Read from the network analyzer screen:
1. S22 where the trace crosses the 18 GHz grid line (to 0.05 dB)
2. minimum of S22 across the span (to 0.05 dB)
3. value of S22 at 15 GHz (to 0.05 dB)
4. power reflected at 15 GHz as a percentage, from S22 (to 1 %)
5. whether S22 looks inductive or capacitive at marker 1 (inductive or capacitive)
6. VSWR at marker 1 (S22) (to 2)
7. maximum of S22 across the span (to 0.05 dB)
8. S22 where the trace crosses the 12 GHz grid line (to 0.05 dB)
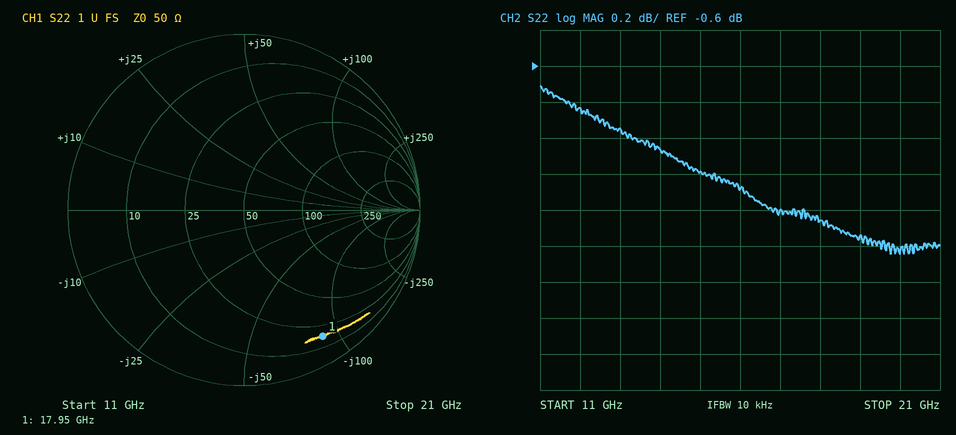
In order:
-1.45 dB
-1.65 dB
-1.20 dB
76 %
capacitive
12
-0.70 dB
-0.85 dB
